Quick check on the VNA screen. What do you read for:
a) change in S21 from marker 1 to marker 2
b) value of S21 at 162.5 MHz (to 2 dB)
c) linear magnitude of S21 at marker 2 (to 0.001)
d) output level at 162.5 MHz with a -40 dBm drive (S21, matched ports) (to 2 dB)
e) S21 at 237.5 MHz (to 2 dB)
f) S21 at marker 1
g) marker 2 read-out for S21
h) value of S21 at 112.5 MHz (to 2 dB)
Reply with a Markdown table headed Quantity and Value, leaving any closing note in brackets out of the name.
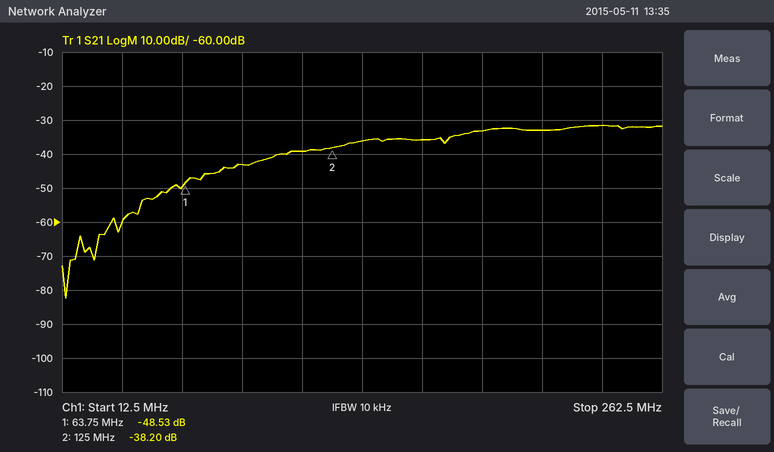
| Quantity | Value |
|---|---|
| change in S21 from marker 1 to marker 2 | 10.33 dB |
| value of S21 at 162.5 MHz | -36 dB |
| linear magnitude of S21 at marker 2 | 0.012 |
| output level at 162.5 MHz with a -40 dBm drive (S21, matched ports) | -76 dBm |
| S21 at 237.5 MHz | -32 dB |
| S21 at marker 1 | -48.53 dB |
| marker 2 read-out for S21 | -38.20 dB |
| value of S21 at 112.5 MHz | -40 dB |
